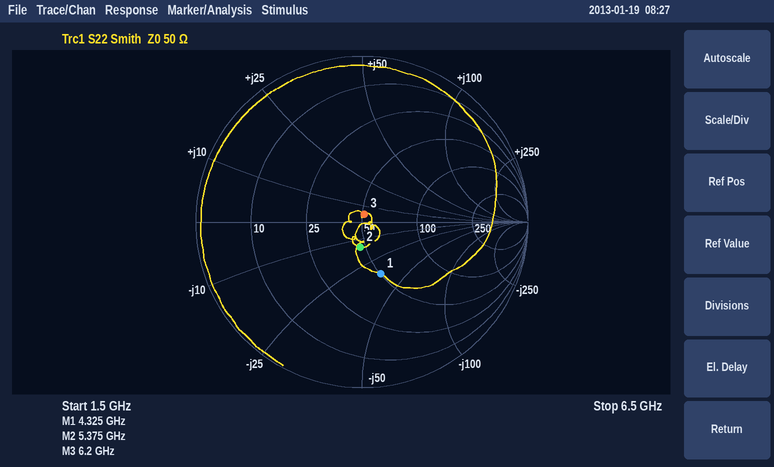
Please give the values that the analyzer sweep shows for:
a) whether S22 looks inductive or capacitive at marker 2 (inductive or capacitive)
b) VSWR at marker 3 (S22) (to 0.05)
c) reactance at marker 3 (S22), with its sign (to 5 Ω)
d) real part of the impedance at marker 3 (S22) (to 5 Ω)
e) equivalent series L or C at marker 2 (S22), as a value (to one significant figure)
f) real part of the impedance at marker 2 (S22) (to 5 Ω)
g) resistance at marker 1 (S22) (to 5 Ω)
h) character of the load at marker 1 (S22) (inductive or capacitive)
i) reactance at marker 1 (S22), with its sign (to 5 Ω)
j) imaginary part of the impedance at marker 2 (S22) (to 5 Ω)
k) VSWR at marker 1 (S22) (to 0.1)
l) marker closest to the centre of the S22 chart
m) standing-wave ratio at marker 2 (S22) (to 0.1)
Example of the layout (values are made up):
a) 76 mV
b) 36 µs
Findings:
a) capacitive
b) 1.10
c) +5 Ω
d) 50 Ω
e) 2 pF
f) 45 Ω
g) 50 Ω
h) capacitive
i) -35 Ω
j) -15 Ω
k) 2.0
l) marker 3
m) 1.4
